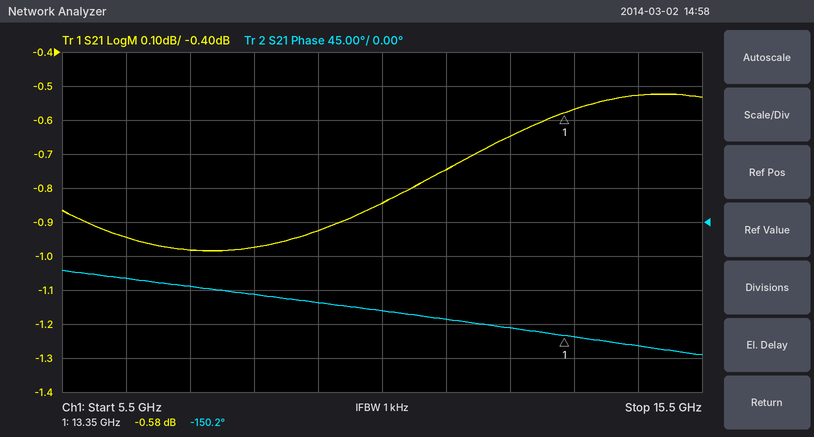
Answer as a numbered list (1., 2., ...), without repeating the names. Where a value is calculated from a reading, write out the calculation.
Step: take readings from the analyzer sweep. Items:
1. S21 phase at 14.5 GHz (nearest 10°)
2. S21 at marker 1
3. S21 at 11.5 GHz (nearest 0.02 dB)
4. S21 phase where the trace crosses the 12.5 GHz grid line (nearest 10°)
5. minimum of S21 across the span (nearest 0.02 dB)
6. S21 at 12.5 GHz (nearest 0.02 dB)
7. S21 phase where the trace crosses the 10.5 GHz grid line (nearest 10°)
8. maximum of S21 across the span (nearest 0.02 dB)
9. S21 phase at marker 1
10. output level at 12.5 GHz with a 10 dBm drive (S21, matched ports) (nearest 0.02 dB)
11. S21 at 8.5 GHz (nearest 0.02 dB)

1. -160°
2. -0.58 dB
3. -0.74 dB
4. -140°
5. -0.98 dB
6. -0.64 dB
7. -120°
8. -0.52 dB
9. -150.2°
10. 10 dBm + (-0.64 dB) = 9.36 dBm
11. -0.98 dB
